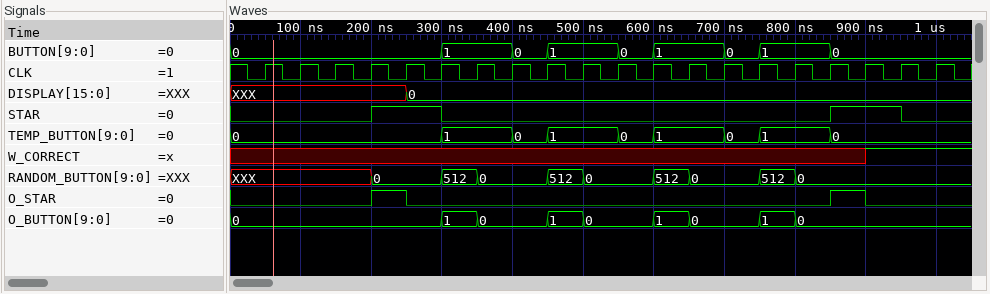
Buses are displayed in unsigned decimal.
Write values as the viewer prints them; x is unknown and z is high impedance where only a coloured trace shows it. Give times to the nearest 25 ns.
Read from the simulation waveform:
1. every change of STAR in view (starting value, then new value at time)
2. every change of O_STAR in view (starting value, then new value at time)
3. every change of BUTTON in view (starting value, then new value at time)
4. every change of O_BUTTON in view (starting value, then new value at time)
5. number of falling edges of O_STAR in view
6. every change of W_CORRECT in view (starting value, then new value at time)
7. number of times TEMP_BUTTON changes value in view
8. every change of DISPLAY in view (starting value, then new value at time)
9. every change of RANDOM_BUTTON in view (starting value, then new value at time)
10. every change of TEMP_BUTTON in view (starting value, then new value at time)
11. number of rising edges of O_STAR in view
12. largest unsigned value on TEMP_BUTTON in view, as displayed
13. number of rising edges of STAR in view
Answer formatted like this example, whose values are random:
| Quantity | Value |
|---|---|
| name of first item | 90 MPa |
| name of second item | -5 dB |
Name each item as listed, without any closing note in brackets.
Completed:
| Quantity | Value |
|---|---|
| every change of STAR in view | 0, 1 at 200 ns, 0 at 300 ns, 1 at 850 ns, 0 at 950 ns |
| every change of O_STAR in view | 0, 1 at 200 ns, 0 at 250 ns, 1 at 850 ns, 0 at 900 ns |
| every change of BUTTON in view | 0, 1 at 300 ns, 0 at 400 ns, 1 at 450 ns, 0 at 550 ns, 1 at 600 ns, 0 at 700 ns, 1 at 750 ns, 0 at 850 ns |
| every change of O_BUTTON in view | 0, 1 at 300 ns, 0 at 350 ns, 1 at 450 ns, 0 at 500 ns, 1 at 600 ns, 0 at 650 ns, 1 at 750 ns, 0 at 800 ns |
| number of falling edges of O_STAR in view | 2 |
| every change of W_CORRECT in view | x, 1 at 900 ns |
| number of times TEMP_BUTTON changes value in view | 8 |
| every change of DISPLAY in view | XXX, 0 at 250 ns |
| every change of RANDOM_BUTTON in view | XXX, 0 at 200 ns, 512 at 300 ns, 0 at 350 ns, 512 at 450 ns, 0 at 500 ns, 512 at 600 ns, 0 at 650 ns, 512 at 750 ns, 0 at 800 ns |
| every change of TEMP_BUTTON in view | 0, 1 at 300 ns, 0 at 400 ns, 1 at 450 ns, 0 at 550 ns, 1 at 600 ns, 0 at 700 ns, 1 at 750 ns, 0 at 850 ns |
| number of rising edges of O_STAR in view | 2 |
| largest unsigned value on TEMP_BUTTON in view, as displayed | 1 |
| number of rising edges of STAR in view | 2 |
